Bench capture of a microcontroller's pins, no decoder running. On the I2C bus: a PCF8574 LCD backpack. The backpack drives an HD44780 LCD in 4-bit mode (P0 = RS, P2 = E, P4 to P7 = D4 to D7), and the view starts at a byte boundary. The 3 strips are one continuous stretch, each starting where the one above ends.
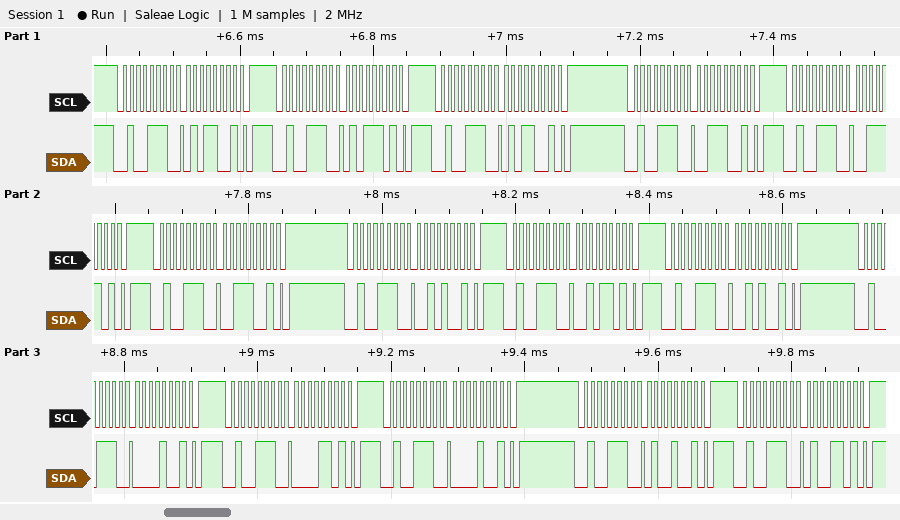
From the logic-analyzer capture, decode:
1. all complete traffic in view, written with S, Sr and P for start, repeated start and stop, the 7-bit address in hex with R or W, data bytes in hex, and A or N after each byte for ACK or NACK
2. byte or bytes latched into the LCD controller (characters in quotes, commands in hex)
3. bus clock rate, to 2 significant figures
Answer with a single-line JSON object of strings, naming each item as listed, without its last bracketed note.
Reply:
{"all complete traffic in view, written with S, Sr and P for start, repeated start and stop, the 7-bit address in hex with R or W, data bytes in hex, and A or N after each byte for ACK or NACK": "S 27W A 59 A P S 27W A 5D A P S 27W A 59 A P S 27W A 39 A P S 27W A 3D A P S 27W A 39 A P S 27W A 29 A P S 27W A 2D A P S 27W A 29 A P S 27W A 09 A P S 27W A 0D A P S 27W A 09 A P S 27W A 49 A P S 27W A 4D A P", "byte or bytes latched into the LCD controller": "'S' ' '", "bus clock rate, to 2 significant figures": "100 kHz"}
